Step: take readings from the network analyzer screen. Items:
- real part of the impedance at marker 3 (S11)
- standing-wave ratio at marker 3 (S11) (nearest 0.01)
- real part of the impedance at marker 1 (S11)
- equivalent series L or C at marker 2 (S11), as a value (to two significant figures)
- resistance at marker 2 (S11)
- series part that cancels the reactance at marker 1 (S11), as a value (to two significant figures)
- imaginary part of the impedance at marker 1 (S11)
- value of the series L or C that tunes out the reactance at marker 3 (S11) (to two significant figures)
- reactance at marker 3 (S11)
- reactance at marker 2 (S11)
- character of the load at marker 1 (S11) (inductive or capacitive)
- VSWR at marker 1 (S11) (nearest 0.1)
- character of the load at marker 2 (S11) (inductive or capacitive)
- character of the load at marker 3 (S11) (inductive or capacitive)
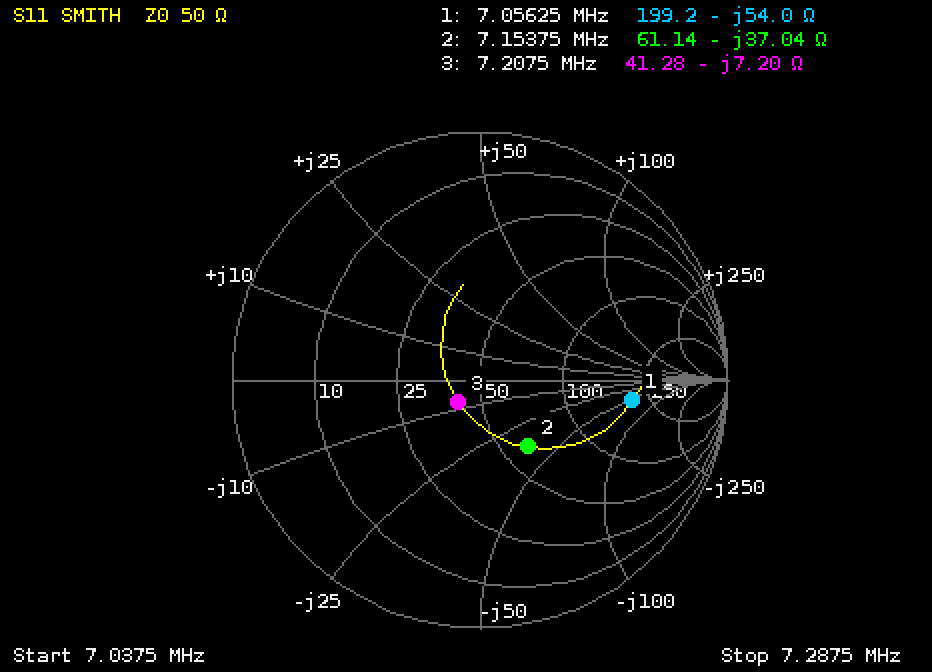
41.28 Ω
1.28
199.2 Ω
600 pF
61.14 Ω
1.2 µH
-54.0 Ω
160 nH
-7.20 Ω
-37.04 Ω
capacitive
4.3
capacitive
capacitive
